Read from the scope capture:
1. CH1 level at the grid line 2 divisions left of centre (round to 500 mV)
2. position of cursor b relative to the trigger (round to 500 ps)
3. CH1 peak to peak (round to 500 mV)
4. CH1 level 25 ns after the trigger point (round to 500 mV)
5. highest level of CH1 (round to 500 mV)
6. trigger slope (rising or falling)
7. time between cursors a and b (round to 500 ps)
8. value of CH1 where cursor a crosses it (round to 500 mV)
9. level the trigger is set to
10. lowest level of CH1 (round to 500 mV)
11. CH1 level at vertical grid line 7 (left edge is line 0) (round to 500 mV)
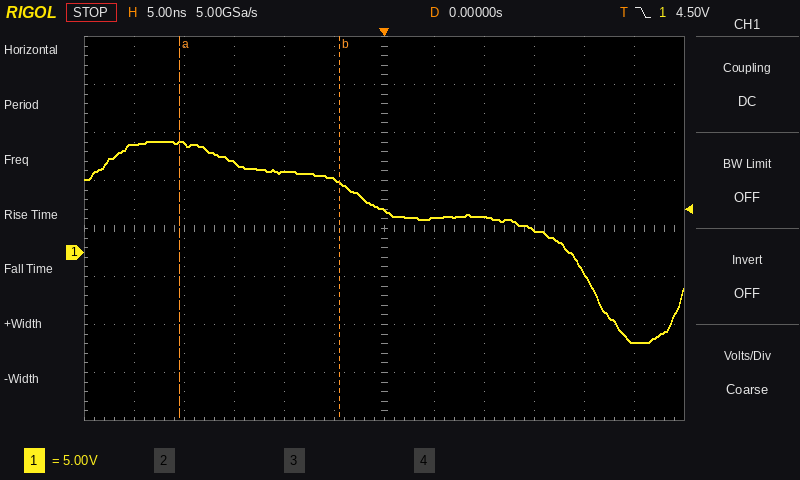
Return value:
8.5 V
-4.5 ns
21.0 V
-9.5 V
11.5 V
falling
16.0 ns
11.5 V
4.50 V
-9.5 V
3.5 V
